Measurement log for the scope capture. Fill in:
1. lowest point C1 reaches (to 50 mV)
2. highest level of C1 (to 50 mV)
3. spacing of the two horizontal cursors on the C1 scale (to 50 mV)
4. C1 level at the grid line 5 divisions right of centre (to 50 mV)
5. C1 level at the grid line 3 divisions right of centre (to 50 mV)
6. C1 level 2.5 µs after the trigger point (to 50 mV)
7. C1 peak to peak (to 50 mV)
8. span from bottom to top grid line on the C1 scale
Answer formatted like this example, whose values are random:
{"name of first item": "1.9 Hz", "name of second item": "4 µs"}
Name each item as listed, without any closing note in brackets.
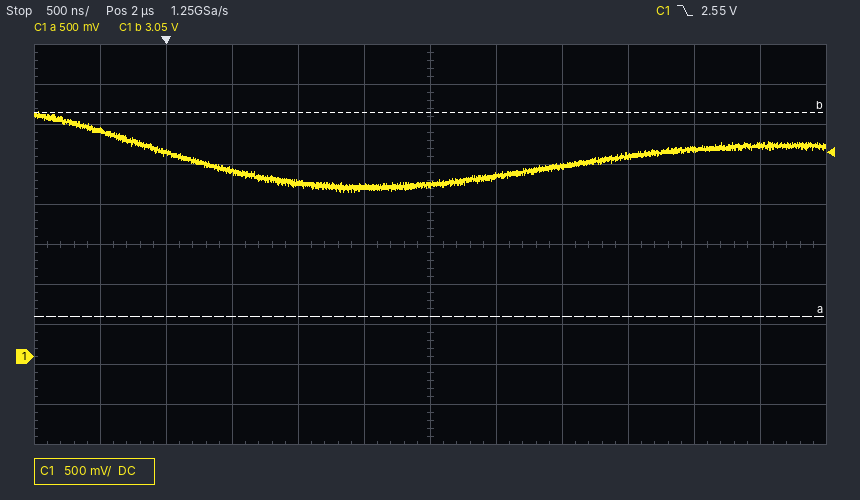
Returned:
{"lowest point C1 reaches": "2.05 V", "highest level of C1": "3.05 V", "spacing of the two horizontal cursors on the C1 scale": "2.55 V", "C1 level at the grid line 5 divisions right of centre": "2.65 V", "C1 level at the grid line 3 divisions right of centre": "2.50 V", "C1 level 2.5 µs after the trigger point": "2.25 V", "C1 peak to peak": "1.00 V", "span from bottom to top grid line on the C1 scale": "5 V"}
